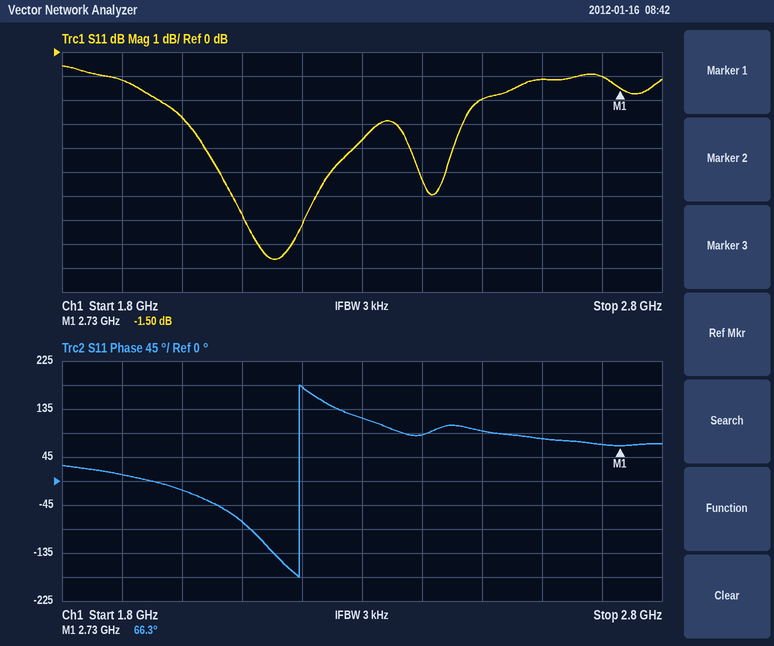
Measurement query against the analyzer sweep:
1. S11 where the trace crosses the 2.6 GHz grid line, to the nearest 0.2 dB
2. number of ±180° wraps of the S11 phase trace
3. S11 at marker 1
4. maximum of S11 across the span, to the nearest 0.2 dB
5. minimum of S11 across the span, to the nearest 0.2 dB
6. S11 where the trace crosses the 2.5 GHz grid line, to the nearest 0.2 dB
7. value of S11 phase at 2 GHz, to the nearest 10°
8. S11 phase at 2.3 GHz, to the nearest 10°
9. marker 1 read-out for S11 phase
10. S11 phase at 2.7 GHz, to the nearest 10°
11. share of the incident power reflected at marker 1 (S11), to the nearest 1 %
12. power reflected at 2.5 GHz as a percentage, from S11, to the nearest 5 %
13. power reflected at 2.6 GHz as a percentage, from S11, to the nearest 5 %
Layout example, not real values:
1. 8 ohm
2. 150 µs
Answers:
1. -1.2 dB
2. 1
3. -1.50 dB
4. -0.6 dB
5. -8.6 dB
6. -2.0 dB
7. -20°
8. 120°
9. 66.3°
10. 70°
11. 71 %
12. 65 %
13. 75 %
